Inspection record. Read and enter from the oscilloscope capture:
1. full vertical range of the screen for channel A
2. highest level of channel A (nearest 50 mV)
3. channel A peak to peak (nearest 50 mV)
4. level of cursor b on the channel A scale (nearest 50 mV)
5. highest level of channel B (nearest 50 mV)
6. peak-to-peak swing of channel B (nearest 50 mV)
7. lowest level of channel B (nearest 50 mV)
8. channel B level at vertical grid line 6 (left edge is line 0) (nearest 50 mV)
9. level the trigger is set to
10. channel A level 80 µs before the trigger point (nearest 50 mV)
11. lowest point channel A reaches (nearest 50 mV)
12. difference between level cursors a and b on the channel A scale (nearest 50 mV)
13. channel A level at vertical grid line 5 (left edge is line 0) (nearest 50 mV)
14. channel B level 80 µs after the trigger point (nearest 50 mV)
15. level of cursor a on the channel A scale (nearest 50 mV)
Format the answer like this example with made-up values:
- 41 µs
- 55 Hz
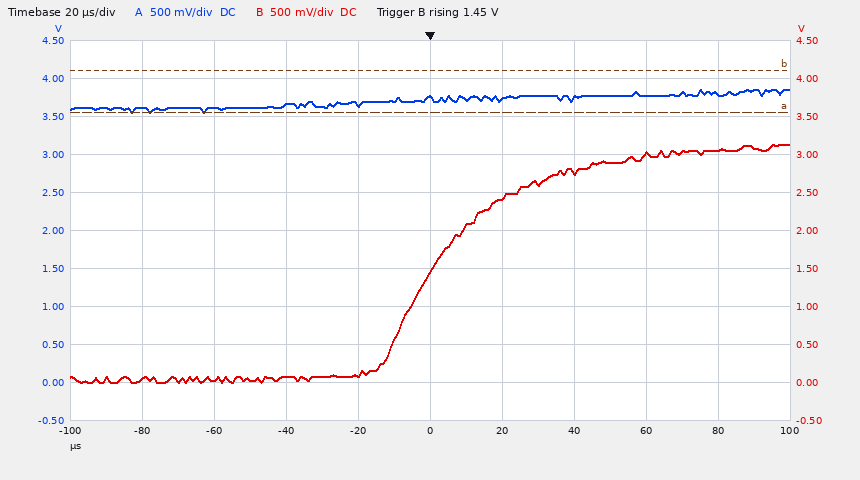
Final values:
- 5 V
- 3.85 V
- 300 mV
- 4.10 V
- 3.15 V
- 3.15 V
- 0 mV
- 2.45 V
- 1.45 V
- 3.60 V
- 3.55 V
- 550 mV
- 3.75 V
- 3.05 V
- 3.55 V
